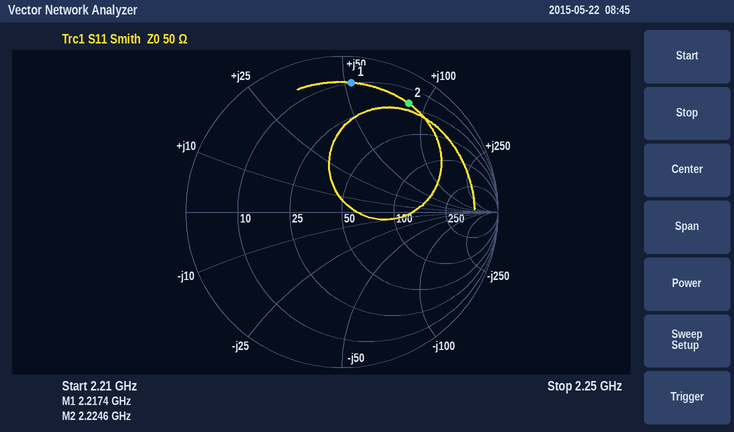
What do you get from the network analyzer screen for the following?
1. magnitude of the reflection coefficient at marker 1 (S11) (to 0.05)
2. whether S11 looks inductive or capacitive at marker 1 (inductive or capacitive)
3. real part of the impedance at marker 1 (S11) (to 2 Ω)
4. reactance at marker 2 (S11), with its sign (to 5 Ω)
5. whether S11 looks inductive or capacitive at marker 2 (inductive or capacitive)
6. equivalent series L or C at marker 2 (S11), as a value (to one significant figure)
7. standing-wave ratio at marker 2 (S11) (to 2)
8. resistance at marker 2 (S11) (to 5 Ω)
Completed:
0.85
inductive
10 Ω
+85 Ω
inductive
6 nH
10
20 Ω
